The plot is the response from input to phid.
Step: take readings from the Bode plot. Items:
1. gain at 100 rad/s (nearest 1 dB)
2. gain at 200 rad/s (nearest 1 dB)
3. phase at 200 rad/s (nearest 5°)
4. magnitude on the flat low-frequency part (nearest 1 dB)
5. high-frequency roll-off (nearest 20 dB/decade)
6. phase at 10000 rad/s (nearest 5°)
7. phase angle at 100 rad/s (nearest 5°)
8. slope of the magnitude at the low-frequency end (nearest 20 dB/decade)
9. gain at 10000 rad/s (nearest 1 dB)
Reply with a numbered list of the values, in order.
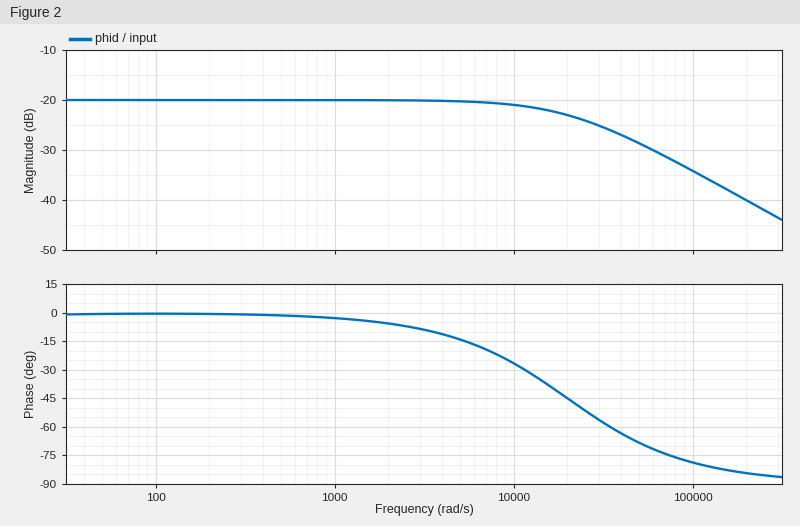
1. -20 dB
2. -20 dB
3. 0°
4. -20 dB
5. -20 dB/decade
6. -25°
7. 0°
8. 0 dB/decade
9. -21 dB
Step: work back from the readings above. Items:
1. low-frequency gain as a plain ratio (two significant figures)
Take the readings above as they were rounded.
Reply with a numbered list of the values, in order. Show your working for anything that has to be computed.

1. 10^(-20 / 20) = 0.10
